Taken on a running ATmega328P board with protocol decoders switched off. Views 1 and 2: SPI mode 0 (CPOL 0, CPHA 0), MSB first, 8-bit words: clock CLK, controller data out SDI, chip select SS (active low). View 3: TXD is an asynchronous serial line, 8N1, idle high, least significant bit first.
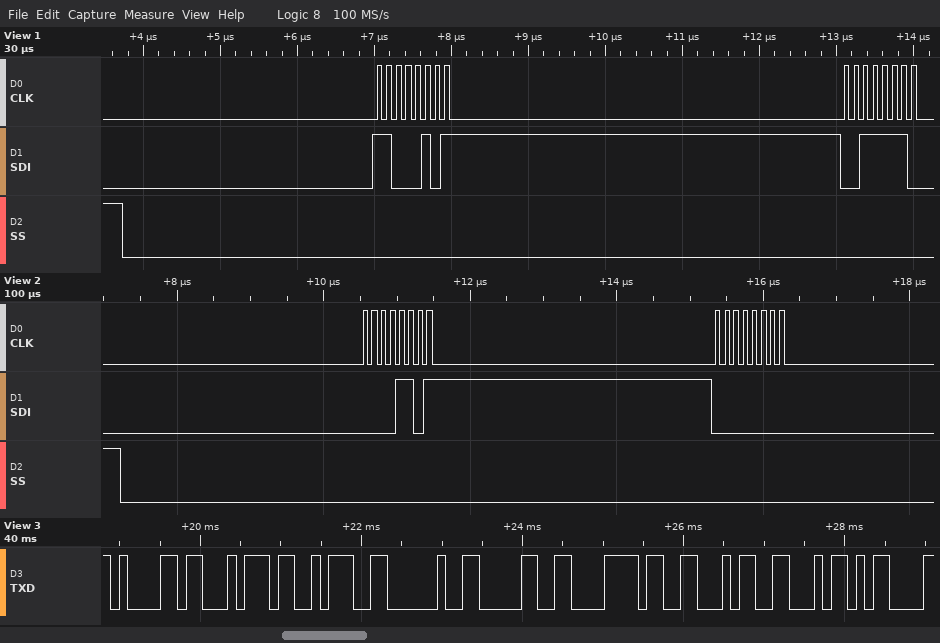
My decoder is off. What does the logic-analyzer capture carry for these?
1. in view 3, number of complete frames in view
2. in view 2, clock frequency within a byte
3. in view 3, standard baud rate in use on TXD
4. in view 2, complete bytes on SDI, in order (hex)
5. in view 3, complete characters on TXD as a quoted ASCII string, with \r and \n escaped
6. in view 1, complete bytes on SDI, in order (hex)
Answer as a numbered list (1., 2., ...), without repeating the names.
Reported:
1. 9
2. 8 MHz
3. 9600 baud
4. 0x0D 0x00
5. "at: 0xFF\r"
6. C5 3E
